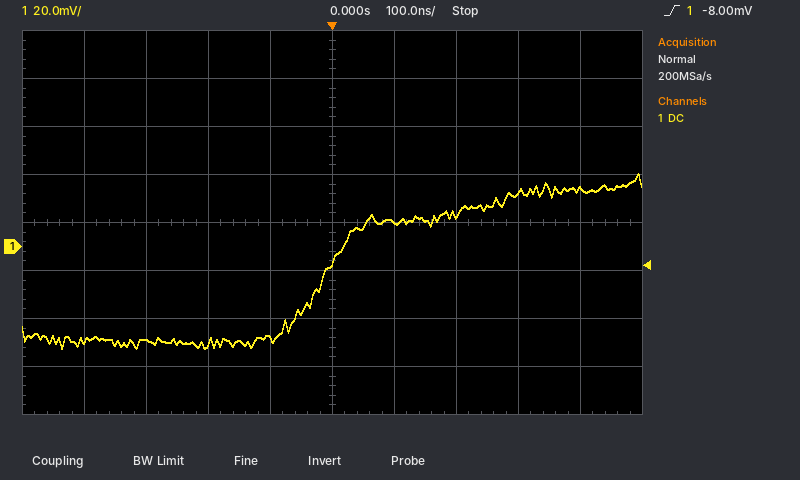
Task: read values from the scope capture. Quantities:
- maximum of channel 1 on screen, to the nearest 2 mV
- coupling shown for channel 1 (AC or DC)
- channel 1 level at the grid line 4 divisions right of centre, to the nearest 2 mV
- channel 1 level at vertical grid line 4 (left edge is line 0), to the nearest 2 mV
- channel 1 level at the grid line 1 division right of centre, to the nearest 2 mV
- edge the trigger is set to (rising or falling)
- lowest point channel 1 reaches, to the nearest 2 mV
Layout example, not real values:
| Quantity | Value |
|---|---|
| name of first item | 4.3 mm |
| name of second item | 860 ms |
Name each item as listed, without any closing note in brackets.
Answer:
| Quantity | Value |
|---|---|
| maximum of channel 1 on screen, to the nearest 2 mV | 30 mV |
| coupling shown for channel 1 | DC |
| channel 1 level at the grid line 4 divisions right of centre, to the nearest 2 mV | 24 mV |
| channel 1 level at vertical grid line 4 (left edge is line 0), to the nearest 2 mV | -38 mV |
| channel 1 level at the grid line 1 division right of centre, to the nearest 2 mV | 10 mV |
| edge the trigger is set to | rising |
| lowest point channel 1 reaches, to the nearest 2 mV | -42 mV |
